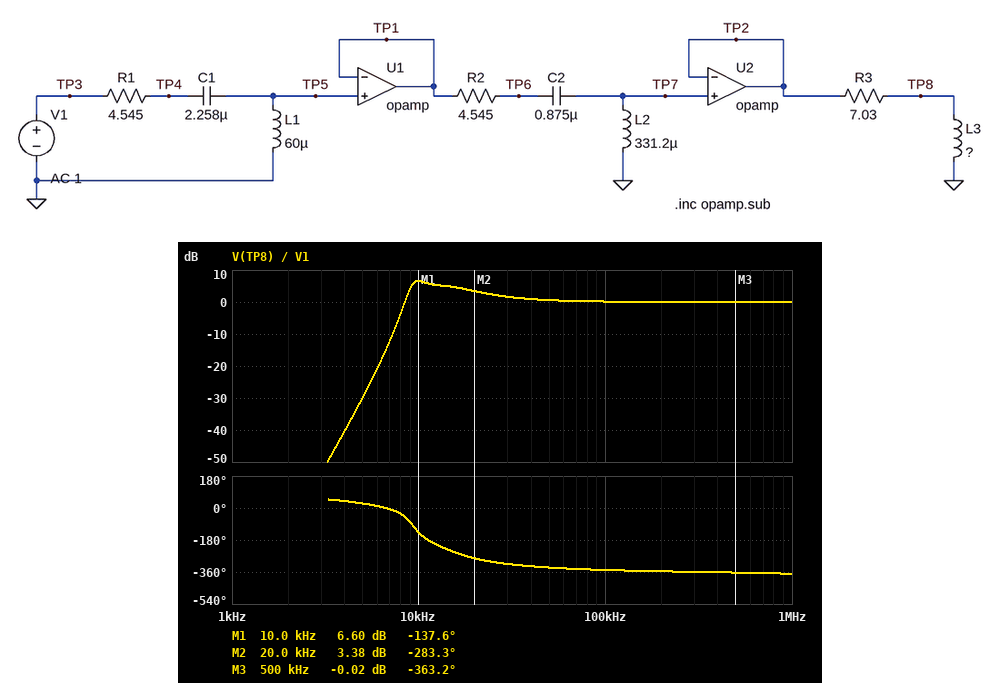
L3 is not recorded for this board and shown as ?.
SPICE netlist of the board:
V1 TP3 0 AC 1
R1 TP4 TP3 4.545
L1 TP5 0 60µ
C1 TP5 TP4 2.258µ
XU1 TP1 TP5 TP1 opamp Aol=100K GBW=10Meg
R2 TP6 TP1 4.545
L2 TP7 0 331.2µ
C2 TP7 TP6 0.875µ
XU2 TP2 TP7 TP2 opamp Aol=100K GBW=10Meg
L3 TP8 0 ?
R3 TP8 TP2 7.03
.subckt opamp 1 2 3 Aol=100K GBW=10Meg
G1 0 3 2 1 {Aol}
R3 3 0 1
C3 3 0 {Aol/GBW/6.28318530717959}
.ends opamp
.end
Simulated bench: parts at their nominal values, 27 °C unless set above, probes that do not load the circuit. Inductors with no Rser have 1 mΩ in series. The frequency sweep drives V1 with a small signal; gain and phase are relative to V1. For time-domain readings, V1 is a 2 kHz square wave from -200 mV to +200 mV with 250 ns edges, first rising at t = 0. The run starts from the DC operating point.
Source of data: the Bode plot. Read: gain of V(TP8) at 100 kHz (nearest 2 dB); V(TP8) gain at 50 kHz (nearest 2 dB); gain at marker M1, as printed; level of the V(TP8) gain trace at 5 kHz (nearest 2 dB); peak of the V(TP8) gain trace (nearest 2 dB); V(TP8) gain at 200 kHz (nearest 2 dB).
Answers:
0 dB
0 dB
6.60 dB
-30 dB
6 dB
0 dB
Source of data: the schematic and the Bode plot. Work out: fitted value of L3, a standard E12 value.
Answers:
150 µH
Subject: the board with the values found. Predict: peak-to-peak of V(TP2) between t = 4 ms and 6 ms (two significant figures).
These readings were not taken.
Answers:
810 mV
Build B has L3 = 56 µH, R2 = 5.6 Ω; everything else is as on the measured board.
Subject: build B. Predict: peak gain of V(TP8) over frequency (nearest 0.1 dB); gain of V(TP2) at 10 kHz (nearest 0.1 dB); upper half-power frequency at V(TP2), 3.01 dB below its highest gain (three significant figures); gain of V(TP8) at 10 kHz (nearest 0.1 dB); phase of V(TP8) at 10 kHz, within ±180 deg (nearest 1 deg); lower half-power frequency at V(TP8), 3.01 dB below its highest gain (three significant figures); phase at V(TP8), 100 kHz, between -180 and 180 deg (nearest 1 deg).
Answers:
1.2 dB
7.1 dB
19.3 kHz
0.1 dB
-106 deg
9.24 kHz
19 deg
